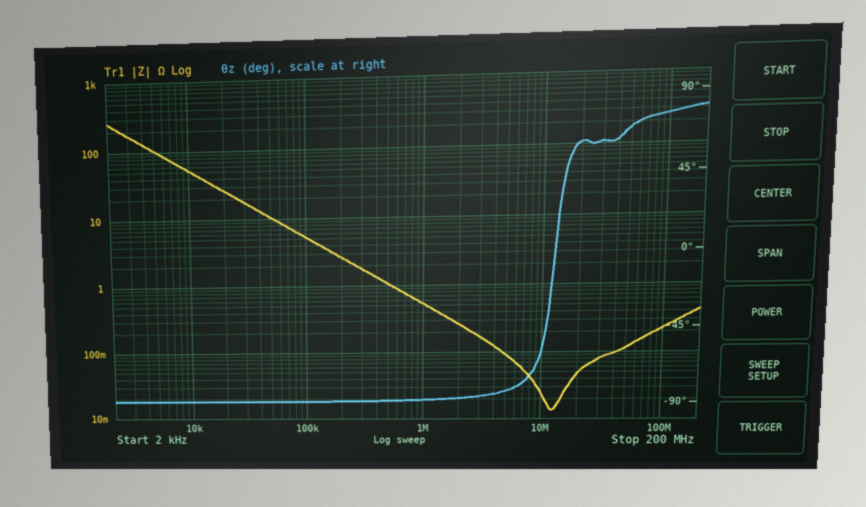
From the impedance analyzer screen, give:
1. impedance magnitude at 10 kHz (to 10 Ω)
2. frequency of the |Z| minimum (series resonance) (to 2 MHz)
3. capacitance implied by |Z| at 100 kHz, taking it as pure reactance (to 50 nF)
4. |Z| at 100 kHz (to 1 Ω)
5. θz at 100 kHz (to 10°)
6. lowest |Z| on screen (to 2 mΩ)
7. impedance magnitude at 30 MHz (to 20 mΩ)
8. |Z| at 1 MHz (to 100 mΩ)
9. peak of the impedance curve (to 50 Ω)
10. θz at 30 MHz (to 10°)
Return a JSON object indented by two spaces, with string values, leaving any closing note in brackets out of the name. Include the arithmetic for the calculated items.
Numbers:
{
  "impedance magnitude at 10 kHz": "50 Ω",
  "frequency of the |Z| minimum (series resonance)": "12 MHz",
  "capacitance implied by |Z| at 100 kHz, taking it as pure reactance": "C = 1/(2π × 100 kHz × 5 Ω) ≈ 318 nF, so 300 nF to the nearest 50 nF",
  "|Z| at 100 kHz": "5 Ω",
  "θz at 100 kHz": "-90°",
  "lowest |Z| on screen": "14 mΩ",
  "impedance magnitude at 30 MHz": "80 mΩ",
  "|Z| at 1 MHz": "500 mΩ",
  "peak of the impedance curve": "250 Ω",
  "θz at 30 MHz": "60°"
}
